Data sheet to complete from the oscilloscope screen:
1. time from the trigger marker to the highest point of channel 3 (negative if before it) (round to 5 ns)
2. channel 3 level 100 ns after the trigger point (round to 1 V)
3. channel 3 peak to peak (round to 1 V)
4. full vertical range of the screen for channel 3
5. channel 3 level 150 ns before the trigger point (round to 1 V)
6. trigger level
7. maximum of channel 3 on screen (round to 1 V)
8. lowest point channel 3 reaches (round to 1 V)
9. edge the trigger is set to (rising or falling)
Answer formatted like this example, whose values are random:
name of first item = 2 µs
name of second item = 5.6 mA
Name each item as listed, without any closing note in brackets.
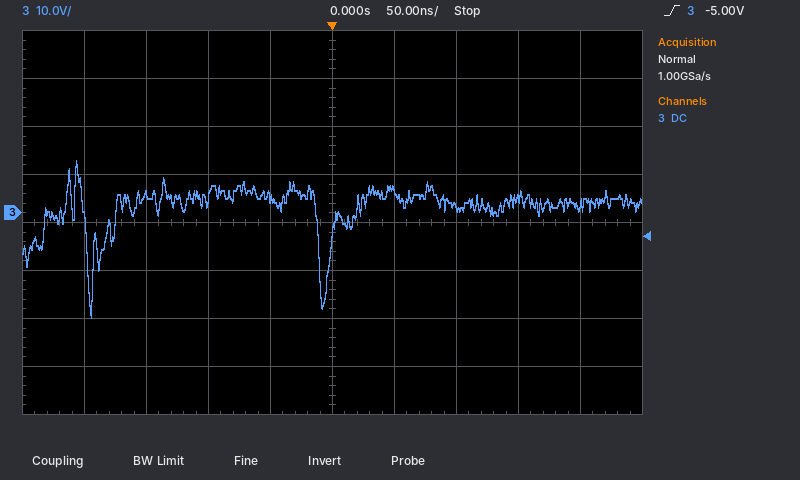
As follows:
time from the trigger marker to the highest point of channel 3 (negative if before it) = -205 ns
channel 3 level 100 ns after the trigger point = 1 V
channel 3 peak to peak = 33 V
full vertical range of the screen for channel 3 = 80 V
channel 3 level 150 ns before the trigger point = 4 V
trigger level = -5.00 V
maximum of channel 3 on screen = 11 V
lowest point channel 3 reaches = -22 V
edge the trigger is set to = rising
